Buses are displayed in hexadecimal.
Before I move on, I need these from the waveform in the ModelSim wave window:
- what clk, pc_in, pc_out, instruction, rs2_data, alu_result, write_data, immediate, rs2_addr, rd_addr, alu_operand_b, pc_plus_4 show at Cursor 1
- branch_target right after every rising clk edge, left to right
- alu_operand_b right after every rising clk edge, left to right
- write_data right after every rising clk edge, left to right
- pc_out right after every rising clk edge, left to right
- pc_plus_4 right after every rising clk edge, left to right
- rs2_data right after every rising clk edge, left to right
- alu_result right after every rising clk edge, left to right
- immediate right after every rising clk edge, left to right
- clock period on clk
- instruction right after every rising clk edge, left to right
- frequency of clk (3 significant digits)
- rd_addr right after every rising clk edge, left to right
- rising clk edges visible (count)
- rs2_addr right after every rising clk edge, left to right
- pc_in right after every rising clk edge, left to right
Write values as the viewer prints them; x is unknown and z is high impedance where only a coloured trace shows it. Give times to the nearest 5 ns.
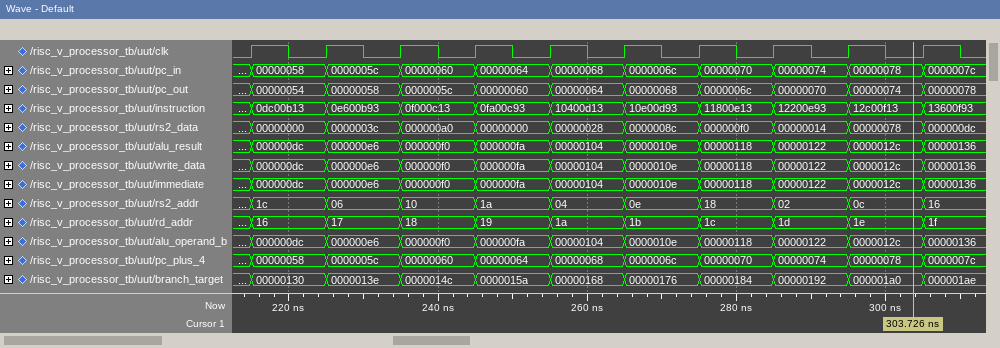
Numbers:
clk=0, pc_in=00000078, pc_out=00000074, instruction=12c00f13, rs2_data=00000078, alu_result=0000012c, write_data=0000012c, immediate=0000012c, rs2_addr=0c, rd_addr=1e, alu_operand_b=0000012c, pc_plus_4=00000078
00000130, 0000013e, 0000014c, 0000015a, 00000168, 00000176, 00000184, 00000192, 000001a0, 000001ae
000000dc, 000000e6, 000000f0, 000000fa, 00000104, 0000010e, 00000118, 00000122, 0000012c, 00000136
000000dc, 000000e6, 000000f0, 000000fa, 00000104, 0000010e, 00000118, 00000122, 0000012c, 00000136
00000054, 00000058, 0000005c, 00000060, 00000064, 00000068, 0000006c, 00000070, 00000074, 00000078
00000058, 0000005c, 00000060, 00000064, 00000068, 0000006c, 00000070, 00000074, 00000078, 0000007c
00000000, 0000003c, 000000a0, 00000000, 00000028, 0000008c, 000000f0, 00000014, 00000078, 000000dc
000000dc, 000000e6, 000000f0, 000000fa, 00000104, 0000010e, 00000118, 00000122, 0000012c, 00000136
000000dc, 000000e6, 000000f0, 000000fa, 00000104, 0000010e, 00000118, 00000122, 0000012c, 00000136
10 ns
0dc00b13, 0e600b93, 0f000c13, 0fa00c93, 10400d13, 10e00d93, 11800e13, 12200e93, 12c00f13, 13600f93
100 MHz
16, 17, 18, 19, 1a, 1b, 1c, 1d, 1e, 1f
10
1c, 06, 10, 1a, 04, 0e, 18, 02, 0c, 16
00000058, 0000005c, 00000060, 00000064, 00000068, 0000006c, 00000070, 00000074, 00000078, 0000007c
